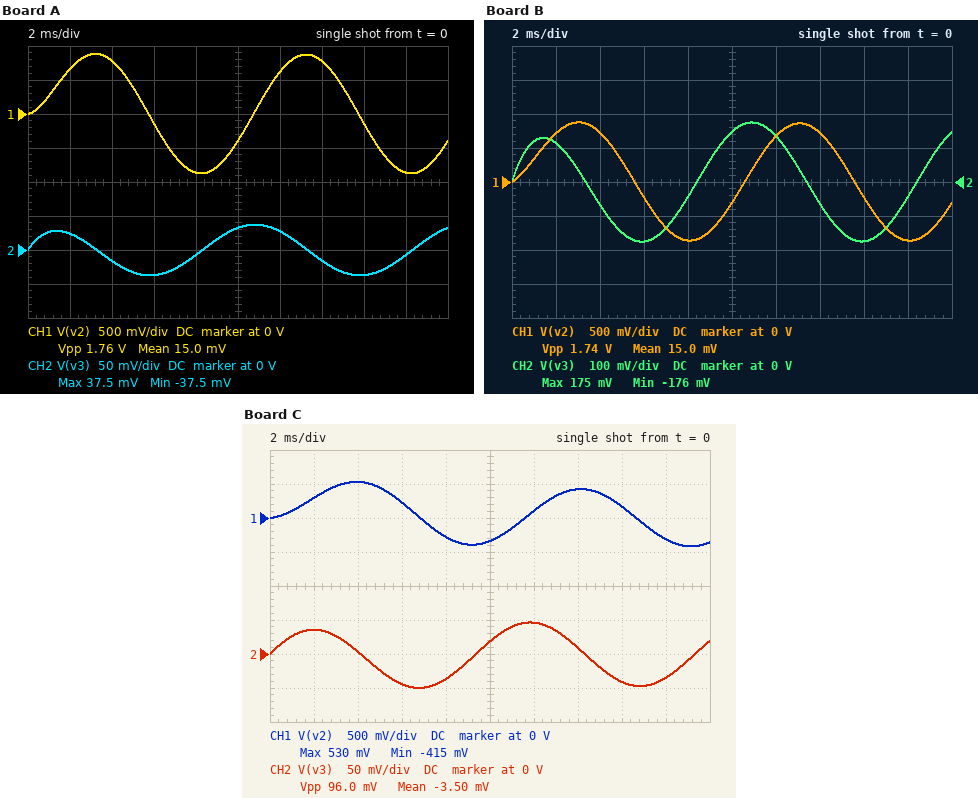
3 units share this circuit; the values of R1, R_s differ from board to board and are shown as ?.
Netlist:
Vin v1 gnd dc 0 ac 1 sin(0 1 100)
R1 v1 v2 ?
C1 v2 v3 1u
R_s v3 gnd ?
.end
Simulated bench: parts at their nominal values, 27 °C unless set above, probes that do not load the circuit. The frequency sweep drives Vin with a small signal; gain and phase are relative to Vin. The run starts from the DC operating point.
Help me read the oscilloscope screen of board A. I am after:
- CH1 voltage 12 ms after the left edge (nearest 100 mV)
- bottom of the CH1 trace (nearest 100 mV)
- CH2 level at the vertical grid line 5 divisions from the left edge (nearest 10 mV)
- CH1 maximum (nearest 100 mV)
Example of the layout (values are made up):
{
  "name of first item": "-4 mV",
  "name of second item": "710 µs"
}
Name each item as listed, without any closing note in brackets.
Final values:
{
  "CH1 voltage 12 ms after the left edge": "600 mV",
  "bottom of the CH1 trace": "-900 mV",
  "CH2 level at the vertical grid line 5 divisions from the left edge": "30 mV",
  "CH1 maximum": "900 mV"
}
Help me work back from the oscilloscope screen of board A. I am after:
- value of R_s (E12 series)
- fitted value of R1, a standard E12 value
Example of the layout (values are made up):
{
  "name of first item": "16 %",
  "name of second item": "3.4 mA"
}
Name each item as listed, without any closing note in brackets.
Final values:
{
  "value of R_s": "68 Ω",
  "fitted value of R1, a standard E12 value": "820 Ω"
}
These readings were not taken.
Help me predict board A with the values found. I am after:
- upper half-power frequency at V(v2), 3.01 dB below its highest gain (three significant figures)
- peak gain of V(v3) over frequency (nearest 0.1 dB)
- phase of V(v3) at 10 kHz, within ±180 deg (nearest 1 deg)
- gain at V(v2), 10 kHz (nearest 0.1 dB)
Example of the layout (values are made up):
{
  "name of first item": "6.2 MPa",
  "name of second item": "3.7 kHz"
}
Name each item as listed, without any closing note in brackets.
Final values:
{
  "upper half-power frequency at V(v2), 3.01 dB below its highest gain": "180 Hz",
  "peak gain of V(v3) over frequency": "-22.3 dB",
  "phase of V(v3) at 10 kHz, within ±180 deg": "1 deg",
  "gain at V(v2), 10 kHz": "-22.1 dB"
}
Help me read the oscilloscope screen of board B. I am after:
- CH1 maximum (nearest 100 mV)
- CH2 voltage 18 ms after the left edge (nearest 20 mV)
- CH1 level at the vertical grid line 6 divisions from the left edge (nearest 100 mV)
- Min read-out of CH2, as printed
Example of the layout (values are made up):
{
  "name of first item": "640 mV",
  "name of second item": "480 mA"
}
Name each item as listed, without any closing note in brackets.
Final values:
{
  "CH1 maximum": "900 mV",
  "CH2 voltage 18 ms after the left edge": "-40 mV",
  "CH1 level at the vertical grid line 6 divisions from the left edge": "700 mV",
  "Min read-out of CH2, as printed": "-176 mV"
}
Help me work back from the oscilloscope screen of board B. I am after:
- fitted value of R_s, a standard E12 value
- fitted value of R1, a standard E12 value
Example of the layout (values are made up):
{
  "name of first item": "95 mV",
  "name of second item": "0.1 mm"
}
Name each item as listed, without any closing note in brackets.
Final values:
{
  "fitted value of R_s, a standard E12 value": "330 Ω",
  "fitted value of R1, a standard E12 value": "680 Ω"
}
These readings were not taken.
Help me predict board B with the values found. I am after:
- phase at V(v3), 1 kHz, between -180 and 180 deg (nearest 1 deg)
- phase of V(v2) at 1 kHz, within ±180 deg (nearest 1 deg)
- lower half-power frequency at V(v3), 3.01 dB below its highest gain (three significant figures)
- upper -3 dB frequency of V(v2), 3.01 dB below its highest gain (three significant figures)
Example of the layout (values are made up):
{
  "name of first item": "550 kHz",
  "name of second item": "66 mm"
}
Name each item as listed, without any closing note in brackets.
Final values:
{
  "phase at V(v3), 1 kHz, between -180 and 180 deg": "9 deg",
  "phase of V(v2) at 1 kHz, within ±180 deg": "-17 deg",
  "lower half-power frequency at V(v3), 3.01 dB below its highest gain": "158 Hz",
  "upper -3 dB frequency of V(v2), 3.01 dB below its highest gain": "178 Hz"
}
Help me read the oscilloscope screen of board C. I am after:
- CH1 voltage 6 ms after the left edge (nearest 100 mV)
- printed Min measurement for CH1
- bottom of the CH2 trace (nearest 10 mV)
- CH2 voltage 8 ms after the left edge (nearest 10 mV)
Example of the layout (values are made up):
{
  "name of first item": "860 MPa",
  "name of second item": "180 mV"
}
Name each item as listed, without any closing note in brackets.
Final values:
{
  "CH1 voltage 6 ms after the left edge": "200 mV",
  "printed Min measurement for CH1": "-415 mV",
  "bottom of the CH2 trace": "-50 mV",
  "CH2 voltage 8 ms after the left edge": "-40 mV"
}
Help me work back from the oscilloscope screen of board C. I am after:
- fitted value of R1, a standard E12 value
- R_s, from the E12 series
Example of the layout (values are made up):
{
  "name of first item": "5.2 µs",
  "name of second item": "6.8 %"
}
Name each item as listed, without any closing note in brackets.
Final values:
{
  "fitted value of R1, a standard E12 value": "3.3 kΩ",
  "R_s, from the E12 series": "180 Ω"
}
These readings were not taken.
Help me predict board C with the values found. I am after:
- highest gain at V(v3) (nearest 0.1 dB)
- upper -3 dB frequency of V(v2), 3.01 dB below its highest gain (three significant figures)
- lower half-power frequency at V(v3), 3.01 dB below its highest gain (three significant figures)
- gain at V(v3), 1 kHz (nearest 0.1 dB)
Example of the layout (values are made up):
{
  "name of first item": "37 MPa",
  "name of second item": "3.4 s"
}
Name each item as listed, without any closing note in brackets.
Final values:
{
  "highest gain at V(v3)": "-25.7 dB",
  "upper -3 dB frequency of V(v2), 3.01 dB below its highest gain": "45.9 Hz",
  "lower half-power frequency at V(v3), 3.01 dB below its highest gain": "45.7 Hz",
  "gain at V(v3), 1 kHz": "-25.7 dB"
}
